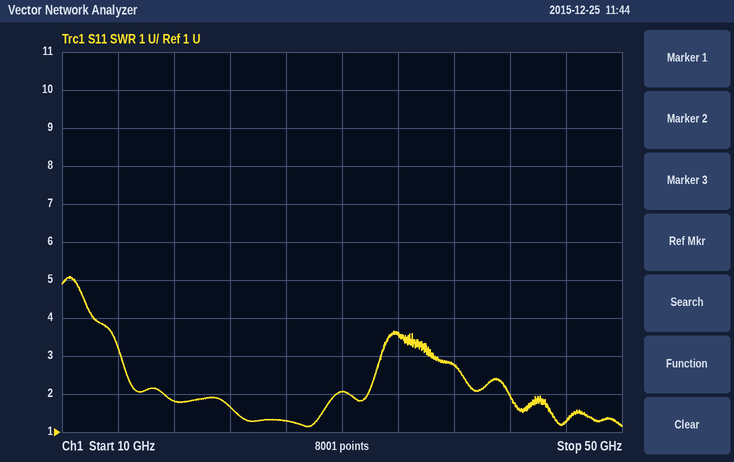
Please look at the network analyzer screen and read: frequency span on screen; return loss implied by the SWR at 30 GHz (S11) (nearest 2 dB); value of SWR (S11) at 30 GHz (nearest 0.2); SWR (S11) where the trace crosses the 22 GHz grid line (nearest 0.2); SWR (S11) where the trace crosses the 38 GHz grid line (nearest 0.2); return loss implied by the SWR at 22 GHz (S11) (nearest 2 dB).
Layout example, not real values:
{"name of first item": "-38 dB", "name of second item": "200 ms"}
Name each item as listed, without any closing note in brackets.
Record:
{"frequency span on screen": "40 GHz", "return loss implied by the SWR at 30 GHz (S11)": "10 dB", "value of SWR (S11) at 30 GHz": "2.0", "SWR (S11) where the trace crosses the 22 GHz grid line": "1.6", "SWR (S11) where the trace crosses the 38 GHz grid line": "2.8", "return loss implied by the SWR at 22 GHz (S11)": "12 dB"}
